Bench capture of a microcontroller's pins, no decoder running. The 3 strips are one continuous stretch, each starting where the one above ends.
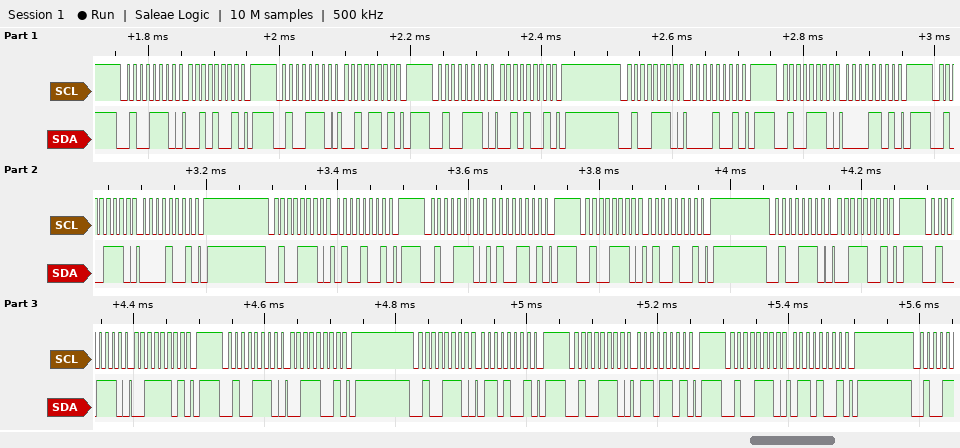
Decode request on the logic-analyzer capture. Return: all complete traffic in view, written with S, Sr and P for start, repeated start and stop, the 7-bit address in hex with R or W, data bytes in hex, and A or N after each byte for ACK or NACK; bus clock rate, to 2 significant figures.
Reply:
S 27W A 29 A P S 27W A 2D A P S 27W A 29 A P S 27W A 09 A P S 27W A 0D A P S 27W A 09 A P S 27W A 49 A P S 27W A 4D A P S 27W A 49 A P S 27W A 39 A P S 27W A 3D A P S 27W A 39 A P S 27W A 69 A P S 27W A 6D A P S 27W A 69 A P
100 kHz
